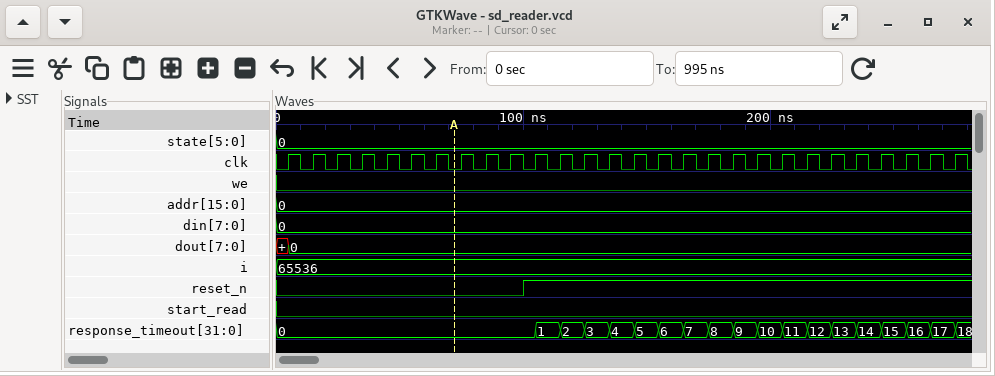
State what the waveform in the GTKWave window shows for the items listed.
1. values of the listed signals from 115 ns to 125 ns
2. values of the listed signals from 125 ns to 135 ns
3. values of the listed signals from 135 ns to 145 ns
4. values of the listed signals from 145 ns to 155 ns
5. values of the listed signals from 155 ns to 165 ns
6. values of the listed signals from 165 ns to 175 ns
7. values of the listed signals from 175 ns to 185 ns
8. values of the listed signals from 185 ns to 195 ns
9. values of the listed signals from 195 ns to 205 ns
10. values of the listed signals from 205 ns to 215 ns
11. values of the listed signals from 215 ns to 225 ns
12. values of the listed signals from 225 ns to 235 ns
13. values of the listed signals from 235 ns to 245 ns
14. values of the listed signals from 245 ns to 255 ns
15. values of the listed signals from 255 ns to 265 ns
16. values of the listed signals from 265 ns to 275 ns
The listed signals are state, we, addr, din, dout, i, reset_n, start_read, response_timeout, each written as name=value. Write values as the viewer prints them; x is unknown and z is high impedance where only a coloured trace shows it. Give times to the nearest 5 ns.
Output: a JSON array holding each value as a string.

["state=0, we=0, addr=0, din=0, dout=0, i=65536, reset_n=1, start_read=0, response_timeout=2", "state=0, we=0, addr=0, din=0, dout=0, i=65536, reset_n=1, start_read=0, response_timeout=3", "state=0, we=0, addr=0, din=0, dout=0, i=65536, reset_n=1, start_read=0, response_timeout=4", "state=0, we=0, addr=0, din=0, dout=0, i=65536, reset_n=1, start_read=0, response_timeout=5", "state=0, we=0, addr=0, din=0, dout=0, i=65536, reset_n=1, start_read=0, response_timeout=6", "state=0, we=0, addr=0, din=0, dout=0, i=65536, reset_n=1, start_read=0, response_timeout=7", "state=0, we=0, addr=0, din=0, dout=0, i=65536, reset_n=1, start_read=0, response_timeout=8", "state=0, we=0, addr=0, din=0, dout=0, i=65536, reset_n=1, start_read=0, response_timeout=9", "state=0, we=0, addr=0, din=0, dout=0, i=65536, reset_n=1, start_read=0, response_timeout=10", "state=0, we=0, addr=0, din=0, dout=0, i=65536, reset_n=1, start_read=0, response_timeout=11", "state=0, we=0, addr=0, din=0, dout=0, i=65536, reset_n=1, start_read=0, response_timeout=12", "state=0, we=0, addr=0, din=0, dout=0, i=65536, reset_n=1, start_read=0, response_timeout=13", "state=0, we=0, addr=0, din=0, dout=0, i=65536, reset_n=1, start_read=0, response_timeout=14", "state=0, we=0, addr=0, din=0, dout=0, i=65536, reset_n=1, start_read=0, response_timeout=15", "state=0, we=0, addr=0, din=0, dout=0, i=65536, reset_n=1, start_read=0, response_timeout=16", "state=0, we=0, addr=0, din=0, dout=0, i=65536, reset_n=1, start_read=0, response_timeout=17"]
